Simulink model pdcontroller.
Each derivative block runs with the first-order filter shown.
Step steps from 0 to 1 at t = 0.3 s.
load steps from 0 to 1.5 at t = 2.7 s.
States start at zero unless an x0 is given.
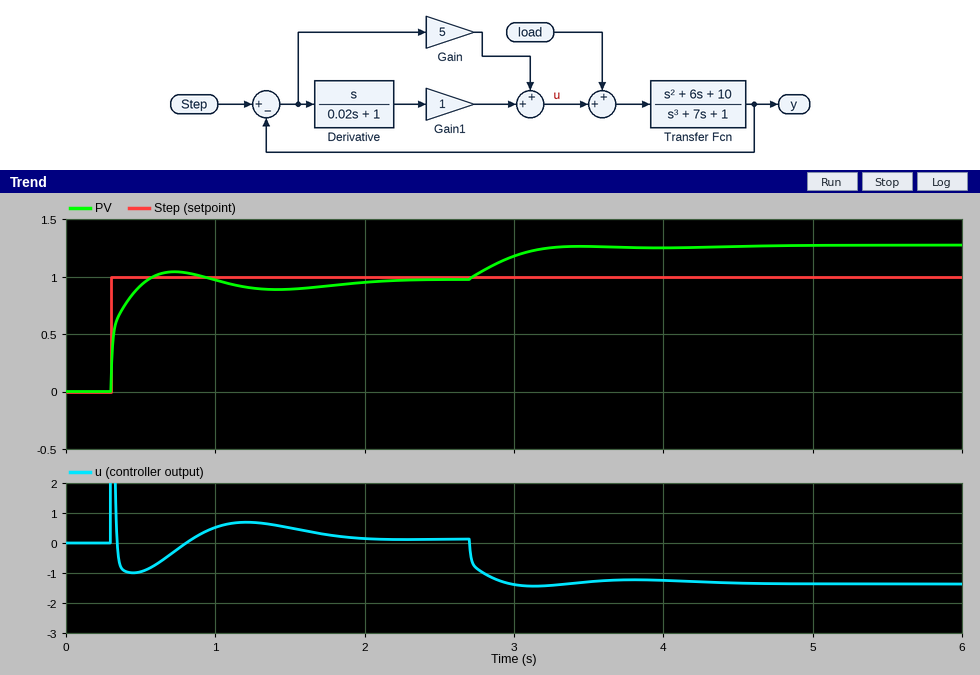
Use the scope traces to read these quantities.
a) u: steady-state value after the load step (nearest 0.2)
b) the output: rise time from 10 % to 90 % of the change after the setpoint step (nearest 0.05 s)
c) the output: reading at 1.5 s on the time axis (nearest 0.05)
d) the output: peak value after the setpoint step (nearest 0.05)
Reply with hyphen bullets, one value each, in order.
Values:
- -1.4
- 0.15 s
- 0.90
- 1.05
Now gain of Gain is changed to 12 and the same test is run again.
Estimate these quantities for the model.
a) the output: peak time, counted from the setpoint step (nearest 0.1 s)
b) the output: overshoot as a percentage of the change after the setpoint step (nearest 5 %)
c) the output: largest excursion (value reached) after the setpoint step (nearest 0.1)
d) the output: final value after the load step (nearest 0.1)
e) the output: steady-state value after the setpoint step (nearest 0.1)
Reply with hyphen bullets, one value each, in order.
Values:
- 0.3 s
- 10 %
- 1.1
- 1.1
- 1.0
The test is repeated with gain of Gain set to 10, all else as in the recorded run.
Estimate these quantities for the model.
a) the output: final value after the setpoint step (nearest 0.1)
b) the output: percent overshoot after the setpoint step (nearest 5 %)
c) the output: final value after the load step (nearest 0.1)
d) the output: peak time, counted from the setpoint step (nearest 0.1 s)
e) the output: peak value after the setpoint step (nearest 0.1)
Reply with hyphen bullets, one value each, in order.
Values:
- 1.0
- 10 %
- 1.1
- 0.3 s
- 1.1
